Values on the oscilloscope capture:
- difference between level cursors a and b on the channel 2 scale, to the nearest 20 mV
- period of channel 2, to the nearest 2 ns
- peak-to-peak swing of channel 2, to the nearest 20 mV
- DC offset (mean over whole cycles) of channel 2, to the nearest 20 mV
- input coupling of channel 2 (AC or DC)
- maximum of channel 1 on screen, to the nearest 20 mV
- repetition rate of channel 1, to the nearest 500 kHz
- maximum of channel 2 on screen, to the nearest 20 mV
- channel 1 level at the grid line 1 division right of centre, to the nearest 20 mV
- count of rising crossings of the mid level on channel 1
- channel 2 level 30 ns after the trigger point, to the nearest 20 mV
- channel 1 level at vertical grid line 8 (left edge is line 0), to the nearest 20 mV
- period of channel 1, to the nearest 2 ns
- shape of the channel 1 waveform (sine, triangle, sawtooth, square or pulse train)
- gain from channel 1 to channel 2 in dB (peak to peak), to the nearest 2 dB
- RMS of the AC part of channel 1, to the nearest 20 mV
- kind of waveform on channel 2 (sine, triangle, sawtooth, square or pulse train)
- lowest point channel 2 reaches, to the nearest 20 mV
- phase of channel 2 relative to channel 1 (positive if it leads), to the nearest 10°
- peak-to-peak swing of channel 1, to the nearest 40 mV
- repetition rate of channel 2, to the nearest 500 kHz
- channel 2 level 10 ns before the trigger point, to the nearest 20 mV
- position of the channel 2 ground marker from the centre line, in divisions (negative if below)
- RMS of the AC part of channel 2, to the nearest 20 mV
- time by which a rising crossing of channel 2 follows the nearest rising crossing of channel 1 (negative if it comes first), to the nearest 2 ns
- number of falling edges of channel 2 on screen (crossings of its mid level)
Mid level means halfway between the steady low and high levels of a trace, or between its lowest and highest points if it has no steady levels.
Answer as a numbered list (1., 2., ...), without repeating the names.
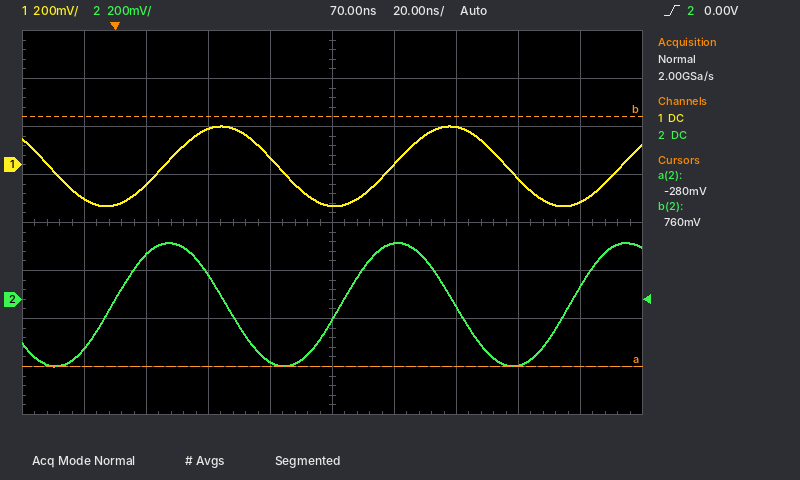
1. 1.04 V
2. 74 ns
3. 520 mV
4. -20 mV
5. DC
6. 160 mV
7. 13.5 MHz
8. 240 mV
9. 0 mV
10. 3
11. 100 mV
12. -60 mV
13. 74 ns
14. sine
15. 4 dB
16. 120 mV
17. sine
18. -280 mV
19. +80°
20. 320 mV
21. 13.5 MHz
22. -200 mV
23. -1.6 div
24. 180 mV
25. -16 ns
26. 2
